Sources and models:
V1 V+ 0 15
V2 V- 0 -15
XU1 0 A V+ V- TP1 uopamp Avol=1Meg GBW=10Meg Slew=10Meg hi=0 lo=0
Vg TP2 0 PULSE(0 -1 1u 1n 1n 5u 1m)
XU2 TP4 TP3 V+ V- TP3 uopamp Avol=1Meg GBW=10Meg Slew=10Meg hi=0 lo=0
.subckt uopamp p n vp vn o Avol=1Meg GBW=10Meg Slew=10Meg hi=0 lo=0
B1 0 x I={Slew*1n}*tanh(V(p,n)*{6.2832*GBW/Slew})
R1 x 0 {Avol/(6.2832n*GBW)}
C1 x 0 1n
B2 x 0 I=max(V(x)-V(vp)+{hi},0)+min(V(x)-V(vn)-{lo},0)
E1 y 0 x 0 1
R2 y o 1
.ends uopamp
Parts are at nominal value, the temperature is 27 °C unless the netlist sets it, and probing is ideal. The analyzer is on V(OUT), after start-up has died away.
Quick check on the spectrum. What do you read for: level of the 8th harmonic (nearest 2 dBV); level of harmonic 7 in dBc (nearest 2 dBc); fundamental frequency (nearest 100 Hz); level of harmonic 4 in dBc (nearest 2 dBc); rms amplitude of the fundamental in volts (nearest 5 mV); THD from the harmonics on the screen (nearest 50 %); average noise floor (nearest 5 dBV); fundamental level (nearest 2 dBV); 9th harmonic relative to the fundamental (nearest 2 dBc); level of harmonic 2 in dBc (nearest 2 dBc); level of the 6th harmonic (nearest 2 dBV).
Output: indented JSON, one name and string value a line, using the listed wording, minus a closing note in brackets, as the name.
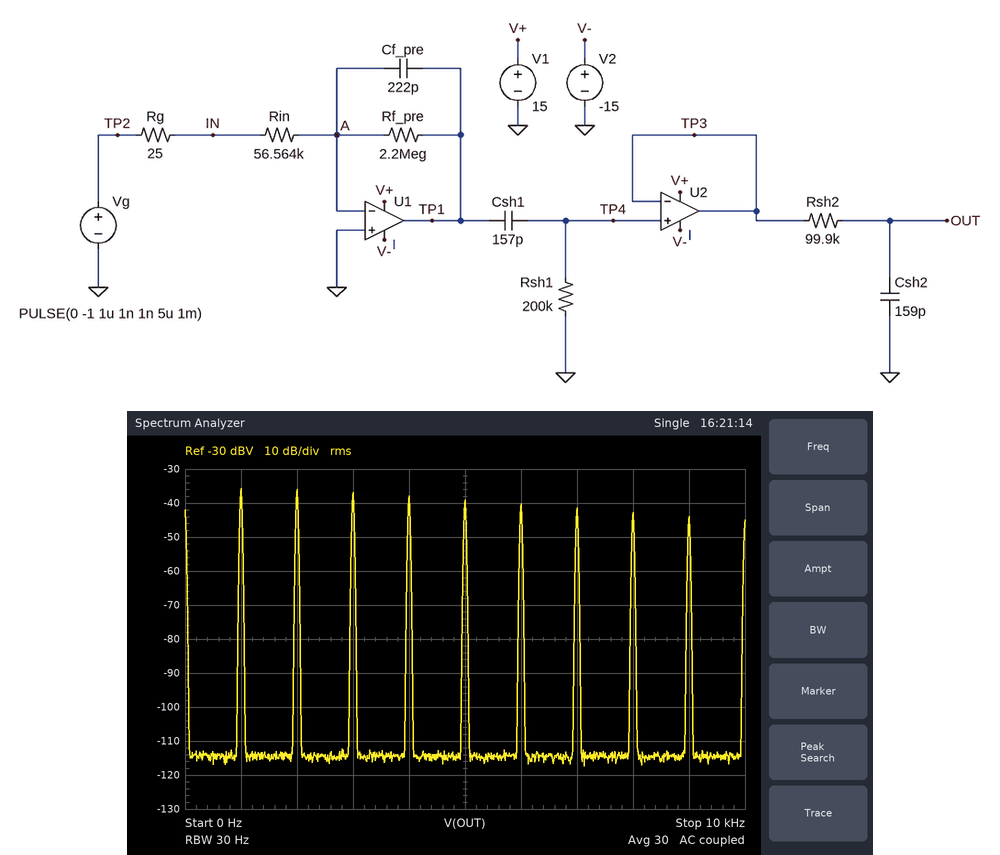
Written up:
{
  "level of the 8th harmonic": "-42 dBV",
  "level of harmonic 7 in dBc": "-6 dBc",
  "fundamental frequency": "1.0 kHz",
  "level of harmonic 4 in dBc": "-2 dBc",
  "rms amplitude of the fundamental in volts": "15 mV",
  "THD from the harmonics on the screen": "200 %",
  "average noise floor": "-115 dBV",
  "fundamental level": "-36 dBV",
  "9th harmonic relative to the fundamental": "-8 dBc",
  "level of harmonic 2 in dBc": "0 dBc",
  "level of the 6th harmonic": "-40 dBV"
}
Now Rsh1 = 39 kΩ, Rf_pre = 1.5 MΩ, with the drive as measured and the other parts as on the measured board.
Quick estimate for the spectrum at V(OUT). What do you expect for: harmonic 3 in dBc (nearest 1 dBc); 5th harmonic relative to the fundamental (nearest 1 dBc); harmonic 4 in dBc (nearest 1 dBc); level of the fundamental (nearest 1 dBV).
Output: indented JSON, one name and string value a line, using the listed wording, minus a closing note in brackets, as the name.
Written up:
{
  "harmonic 3 in dBc": "0 dBc",
  "5th harmonic relative to the fundamental": "0 dBc",
  "harmonic 4 in dBc": "0 dBc",
  "level of the fundamental": "-50 dBV"
}
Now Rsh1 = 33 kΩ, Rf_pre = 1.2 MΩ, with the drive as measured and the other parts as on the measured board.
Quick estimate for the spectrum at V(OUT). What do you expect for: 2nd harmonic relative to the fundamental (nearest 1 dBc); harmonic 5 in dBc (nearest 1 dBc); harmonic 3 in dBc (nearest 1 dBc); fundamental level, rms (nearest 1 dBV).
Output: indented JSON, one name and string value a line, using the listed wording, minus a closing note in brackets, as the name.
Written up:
{
  "2nd harmonic relative to the fundamental": "1 dBc",
  "harmonic 5 in dBc": "0 dBc",
  "harmonic 3 in dBc": "1 dBc",
  "fundamental level, rms": "-52 dBV"
}
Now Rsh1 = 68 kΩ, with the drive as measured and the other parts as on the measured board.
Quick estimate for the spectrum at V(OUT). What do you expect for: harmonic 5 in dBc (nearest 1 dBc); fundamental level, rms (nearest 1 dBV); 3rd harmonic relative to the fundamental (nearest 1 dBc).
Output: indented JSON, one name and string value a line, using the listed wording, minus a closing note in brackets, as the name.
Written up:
{
  "harmonic 5 in dBc": "-1 dBc",
  "fundamental level, rms": "-45 dBV",
  "3rd harmonic relative to the fundamental": "0 dBc"
}
